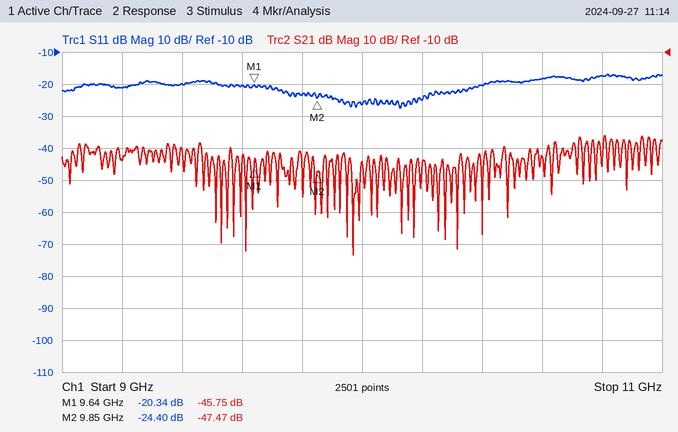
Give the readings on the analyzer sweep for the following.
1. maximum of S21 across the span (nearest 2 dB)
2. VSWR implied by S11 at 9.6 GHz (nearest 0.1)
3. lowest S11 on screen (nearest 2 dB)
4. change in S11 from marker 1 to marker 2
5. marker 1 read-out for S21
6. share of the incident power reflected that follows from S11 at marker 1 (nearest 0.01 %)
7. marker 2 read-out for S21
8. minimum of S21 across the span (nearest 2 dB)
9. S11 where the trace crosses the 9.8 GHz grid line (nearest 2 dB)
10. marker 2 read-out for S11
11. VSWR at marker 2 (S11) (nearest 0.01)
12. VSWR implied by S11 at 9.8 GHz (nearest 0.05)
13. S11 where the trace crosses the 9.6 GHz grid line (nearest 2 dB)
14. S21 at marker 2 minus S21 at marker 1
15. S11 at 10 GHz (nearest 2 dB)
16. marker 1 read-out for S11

-36 dB
1.2
-28 dB
-4.06 dB
-45.75 dB
0.92 %
-47.47 dB
-74 dB
-24 dB
-24.40 dB
1.13
1.15
-20 dB
-1.72 dB
-26 dB
-20.34 dB
